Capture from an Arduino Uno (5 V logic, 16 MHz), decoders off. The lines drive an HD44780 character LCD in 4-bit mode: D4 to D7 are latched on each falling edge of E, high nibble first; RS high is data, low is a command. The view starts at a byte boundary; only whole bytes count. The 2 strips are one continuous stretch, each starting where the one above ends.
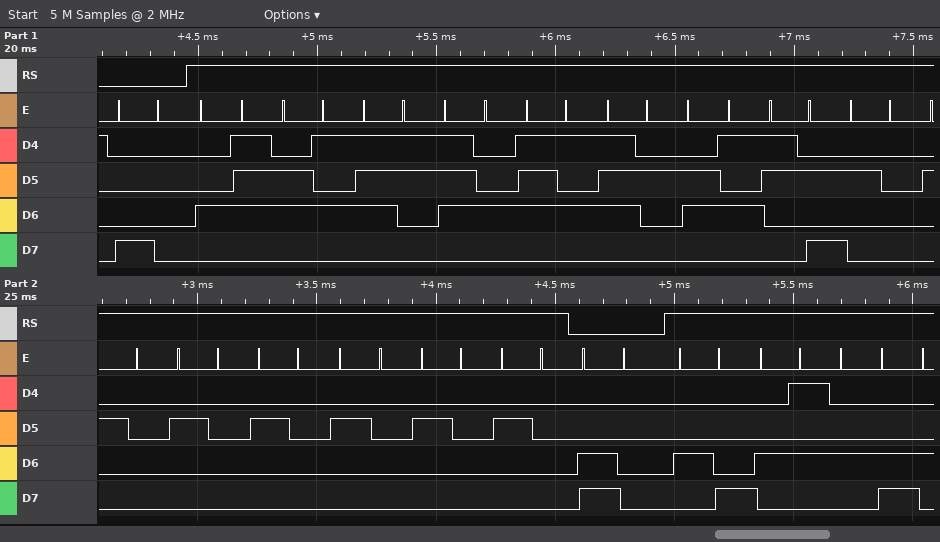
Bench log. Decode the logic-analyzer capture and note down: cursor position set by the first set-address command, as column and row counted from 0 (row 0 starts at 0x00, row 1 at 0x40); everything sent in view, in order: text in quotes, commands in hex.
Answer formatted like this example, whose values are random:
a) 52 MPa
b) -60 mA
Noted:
a) column 0, row 0
b) 0x80 "Gesture:       " 0xC0 "HEL"
